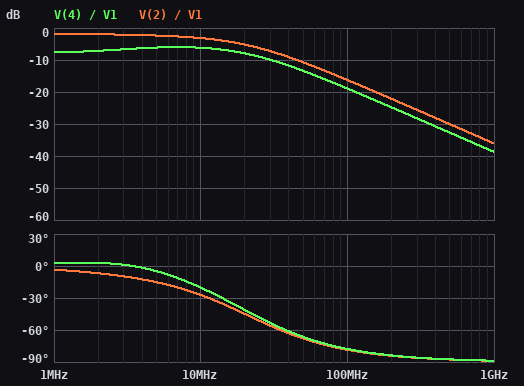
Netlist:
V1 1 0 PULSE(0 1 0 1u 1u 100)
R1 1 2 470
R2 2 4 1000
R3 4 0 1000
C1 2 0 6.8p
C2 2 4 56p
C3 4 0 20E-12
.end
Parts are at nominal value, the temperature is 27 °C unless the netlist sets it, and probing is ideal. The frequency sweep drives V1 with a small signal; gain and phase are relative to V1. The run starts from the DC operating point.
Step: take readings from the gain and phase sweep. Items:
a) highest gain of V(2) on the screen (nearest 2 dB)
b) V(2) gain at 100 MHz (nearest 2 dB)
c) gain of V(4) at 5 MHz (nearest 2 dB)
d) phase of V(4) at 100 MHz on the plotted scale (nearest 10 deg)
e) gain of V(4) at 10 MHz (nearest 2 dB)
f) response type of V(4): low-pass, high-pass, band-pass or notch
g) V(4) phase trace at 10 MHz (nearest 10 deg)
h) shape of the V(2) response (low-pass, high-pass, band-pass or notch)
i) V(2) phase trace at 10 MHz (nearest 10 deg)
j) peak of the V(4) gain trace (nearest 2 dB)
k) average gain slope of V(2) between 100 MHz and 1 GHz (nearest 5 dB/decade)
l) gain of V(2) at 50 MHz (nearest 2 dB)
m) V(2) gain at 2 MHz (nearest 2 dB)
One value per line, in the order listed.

-2 dB
-16 dB
-6 dB
-80 deg
-6 dB
low-pass
-20 deg
low-pass
-30 deg
-6 dB
-20 dB/decade
-10 dB
-2 dB
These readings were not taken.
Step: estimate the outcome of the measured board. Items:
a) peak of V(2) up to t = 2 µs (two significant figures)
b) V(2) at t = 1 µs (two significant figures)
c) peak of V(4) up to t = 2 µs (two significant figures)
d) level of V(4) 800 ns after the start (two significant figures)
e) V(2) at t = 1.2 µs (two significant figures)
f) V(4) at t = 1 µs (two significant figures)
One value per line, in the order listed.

810 mV
800 mV
410 mV
330 mV
810 mV
410 mV
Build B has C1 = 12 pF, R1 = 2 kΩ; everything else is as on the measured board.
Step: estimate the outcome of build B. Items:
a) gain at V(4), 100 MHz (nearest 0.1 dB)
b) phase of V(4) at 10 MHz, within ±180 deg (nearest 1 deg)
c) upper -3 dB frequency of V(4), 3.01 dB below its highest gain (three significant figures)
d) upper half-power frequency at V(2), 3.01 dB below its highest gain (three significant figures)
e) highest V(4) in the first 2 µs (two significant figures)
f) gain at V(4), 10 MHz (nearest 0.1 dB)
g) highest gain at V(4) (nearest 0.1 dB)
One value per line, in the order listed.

-33.2 dB
-51 deg
9.46 MHz
5.19 MHz
250 mV
-15.2 dB
-11.9 dB
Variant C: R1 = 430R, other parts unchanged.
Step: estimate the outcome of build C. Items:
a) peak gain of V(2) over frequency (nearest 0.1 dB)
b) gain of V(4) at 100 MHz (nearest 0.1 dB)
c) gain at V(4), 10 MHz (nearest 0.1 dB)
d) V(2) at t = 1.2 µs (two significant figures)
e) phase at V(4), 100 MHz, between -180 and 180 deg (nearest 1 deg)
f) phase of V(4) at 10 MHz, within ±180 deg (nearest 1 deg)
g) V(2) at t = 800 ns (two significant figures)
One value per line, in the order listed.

-1.7 dB
-18.2 dB
-5.9 dB
820 mV
-77 deg
-19 deg
650 mV
